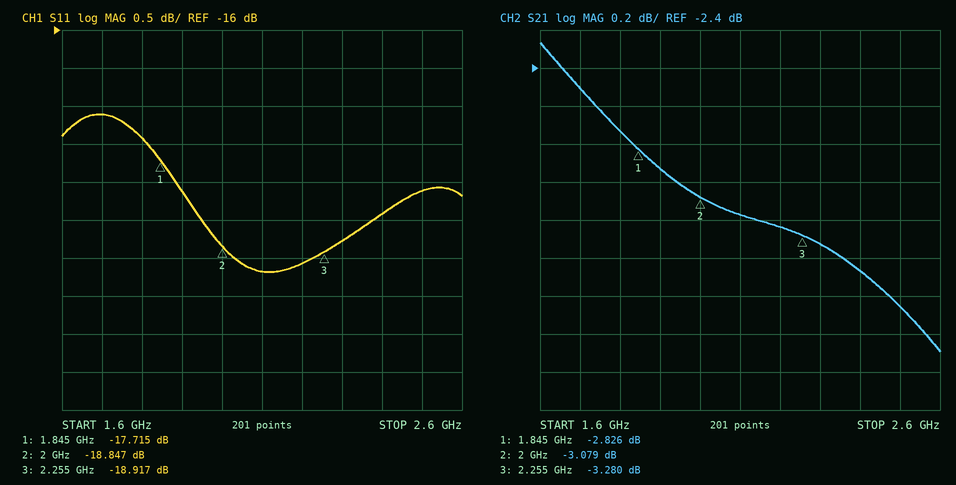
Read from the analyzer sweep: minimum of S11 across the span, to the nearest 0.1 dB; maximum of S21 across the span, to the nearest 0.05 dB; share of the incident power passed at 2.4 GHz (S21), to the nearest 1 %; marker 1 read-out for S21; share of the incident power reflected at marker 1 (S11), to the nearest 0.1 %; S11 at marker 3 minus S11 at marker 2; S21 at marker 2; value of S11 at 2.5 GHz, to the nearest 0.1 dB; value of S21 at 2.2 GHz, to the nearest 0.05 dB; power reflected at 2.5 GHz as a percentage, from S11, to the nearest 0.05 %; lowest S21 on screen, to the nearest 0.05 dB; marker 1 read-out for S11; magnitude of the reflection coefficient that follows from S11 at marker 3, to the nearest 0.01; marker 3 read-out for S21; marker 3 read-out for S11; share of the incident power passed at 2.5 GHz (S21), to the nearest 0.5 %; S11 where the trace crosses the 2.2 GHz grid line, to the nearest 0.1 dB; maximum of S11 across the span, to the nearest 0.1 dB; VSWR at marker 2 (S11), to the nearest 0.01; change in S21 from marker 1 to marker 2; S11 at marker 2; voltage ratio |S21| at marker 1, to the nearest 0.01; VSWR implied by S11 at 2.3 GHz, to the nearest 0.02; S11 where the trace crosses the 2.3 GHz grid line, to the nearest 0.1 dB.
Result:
-19.2 dB
-2.25 dB
45 %
-2.826 dB
1.7 %
-0.070 dB
-3.079 dB
-18.1 dB
-3.25 dB
1.55 %
-3.90 dB
-17.715 dB
0.11
-3.280 dB
-18.917 dB
43.0 %
-19.1 dB
-17.1 dB
1.26
-0.253 dB
-18.847 dB
0.72
1.26
-18.8 dB
